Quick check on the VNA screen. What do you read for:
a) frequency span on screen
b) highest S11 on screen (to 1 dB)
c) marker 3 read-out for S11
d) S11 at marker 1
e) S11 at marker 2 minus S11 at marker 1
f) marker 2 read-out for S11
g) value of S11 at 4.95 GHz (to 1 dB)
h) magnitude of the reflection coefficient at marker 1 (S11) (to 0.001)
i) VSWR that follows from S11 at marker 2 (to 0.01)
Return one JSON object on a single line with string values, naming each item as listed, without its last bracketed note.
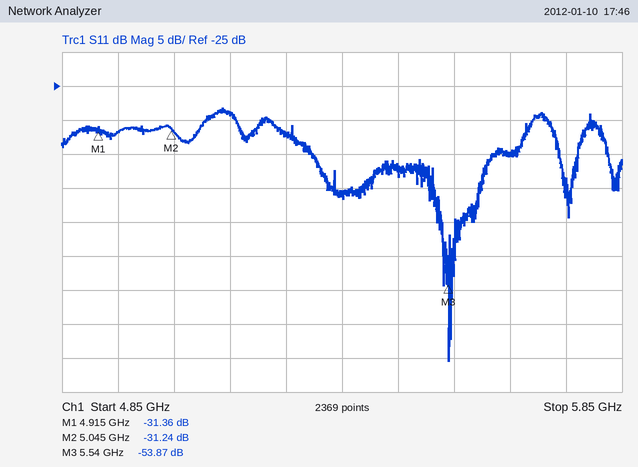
{"frequency span on screen": "1 GHz", "highest S11 on screen": "-28 dB", "marker 3 read-out for S11": "-53.87 dB", "S11 at marker 1": "-31.36 dB", "S11 at marker 2 minus S11 at marker 1": "0.12 dB", "marker 2 read-out for S11": "-31.24 dB", "value of S11 at 4.95 GHz": "-32 dB", "magnitude of the reflection coefficient at marker 1 (S11)": "0.027", "VSWR that follows from S11 at marker 2": "1.06"}
